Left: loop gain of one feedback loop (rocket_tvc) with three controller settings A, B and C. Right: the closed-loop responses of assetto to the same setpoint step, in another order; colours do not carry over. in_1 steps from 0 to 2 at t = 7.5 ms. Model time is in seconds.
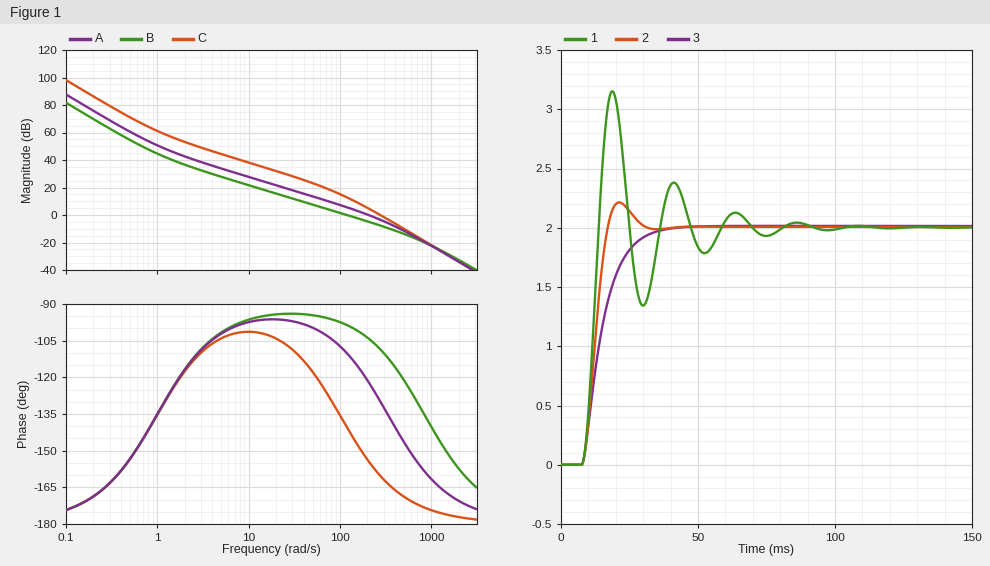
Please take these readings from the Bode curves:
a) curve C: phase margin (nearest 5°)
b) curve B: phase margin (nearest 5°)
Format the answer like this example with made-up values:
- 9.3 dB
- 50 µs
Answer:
- 20°
- 80°
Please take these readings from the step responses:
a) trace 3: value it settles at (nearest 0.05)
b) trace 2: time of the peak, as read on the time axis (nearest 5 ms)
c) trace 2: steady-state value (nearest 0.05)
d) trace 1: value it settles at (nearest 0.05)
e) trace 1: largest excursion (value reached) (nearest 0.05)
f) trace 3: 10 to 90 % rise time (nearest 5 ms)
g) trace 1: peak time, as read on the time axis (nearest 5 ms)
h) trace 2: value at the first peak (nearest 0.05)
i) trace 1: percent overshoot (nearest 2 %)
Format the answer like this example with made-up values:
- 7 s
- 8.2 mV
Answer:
- 2.00
- 20 ms
- 2.00
- 2.00
- 3.15
- 15 ms
- 20 ms
- 2.20
- 58 %
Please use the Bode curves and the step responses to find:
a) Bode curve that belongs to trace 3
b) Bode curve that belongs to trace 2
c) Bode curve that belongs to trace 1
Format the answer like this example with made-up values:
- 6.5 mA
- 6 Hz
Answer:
- B
- A
- C
